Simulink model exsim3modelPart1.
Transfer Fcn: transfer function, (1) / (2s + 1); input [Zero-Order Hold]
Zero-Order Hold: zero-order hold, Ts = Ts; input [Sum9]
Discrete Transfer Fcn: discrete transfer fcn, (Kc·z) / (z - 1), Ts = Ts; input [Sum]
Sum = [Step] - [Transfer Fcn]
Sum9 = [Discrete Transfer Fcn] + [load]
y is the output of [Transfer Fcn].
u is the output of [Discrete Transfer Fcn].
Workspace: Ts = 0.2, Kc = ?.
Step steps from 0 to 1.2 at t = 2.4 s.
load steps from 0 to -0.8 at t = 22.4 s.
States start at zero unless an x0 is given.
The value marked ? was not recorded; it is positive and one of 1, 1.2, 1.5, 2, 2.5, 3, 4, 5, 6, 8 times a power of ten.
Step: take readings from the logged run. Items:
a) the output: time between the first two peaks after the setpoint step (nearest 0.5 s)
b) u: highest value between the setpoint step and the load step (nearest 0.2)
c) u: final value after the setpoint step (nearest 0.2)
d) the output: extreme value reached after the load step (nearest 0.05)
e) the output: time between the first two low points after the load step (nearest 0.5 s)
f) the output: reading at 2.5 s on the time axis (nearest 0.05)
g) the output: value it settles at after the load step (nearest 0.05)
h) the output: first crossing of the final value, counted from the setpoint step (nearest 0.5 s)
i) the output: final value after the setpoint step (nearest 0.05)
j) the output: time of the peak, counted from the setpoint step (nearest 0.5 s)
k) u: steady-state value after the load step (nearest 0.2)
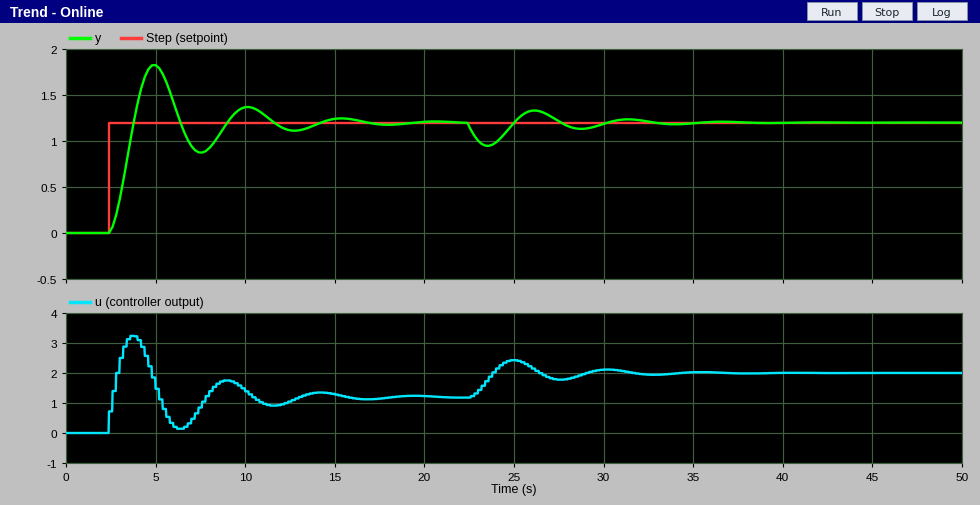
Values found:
5.0 s
3.2
1.2
0.95
5.0 s
0.05
1.20
1.5 s
1.20
2.5 s
2.0
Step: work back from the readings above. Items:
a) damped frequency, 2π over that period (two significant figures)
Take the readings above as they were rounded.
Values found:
1.3 rad/s
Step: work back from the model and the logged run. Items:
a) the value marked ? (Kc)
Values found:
0.6
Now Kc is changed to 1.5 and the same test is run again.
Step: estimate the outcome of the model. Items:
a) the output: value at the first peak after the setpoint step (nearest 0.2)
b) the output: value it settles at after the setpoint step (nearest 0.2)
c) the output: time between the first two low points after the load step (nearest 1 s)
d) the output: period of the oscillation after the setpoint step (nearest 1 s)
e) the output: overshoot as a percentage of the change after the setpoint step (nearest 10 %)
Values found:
2.0
1.2
3 s
3 s
70 %
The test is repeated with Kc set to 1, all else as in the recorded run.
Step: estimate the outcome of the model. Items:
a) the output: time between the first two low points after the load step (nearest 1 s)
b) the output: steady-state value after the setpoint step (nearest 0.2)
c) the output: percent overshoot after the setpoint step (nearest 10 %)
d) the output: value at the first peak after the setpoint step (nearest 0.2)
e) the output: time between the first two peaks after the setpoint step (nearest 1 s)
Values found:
4 s
1.2
60 %
2.0
4 s
